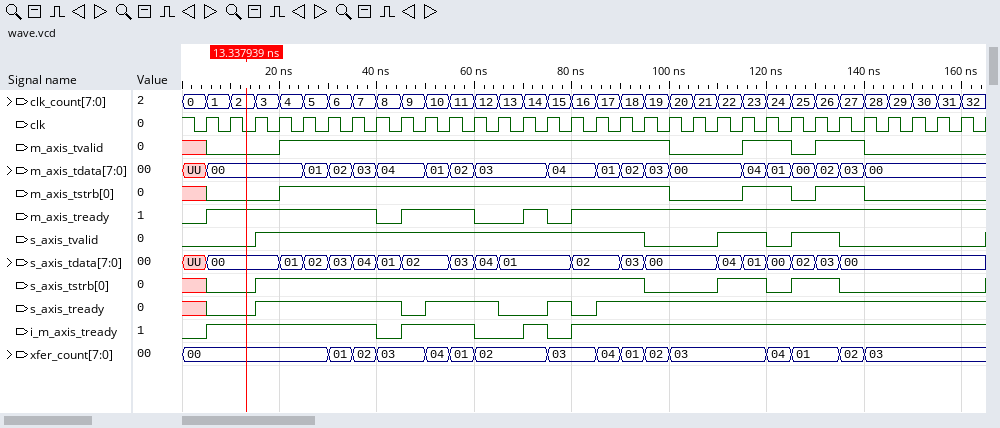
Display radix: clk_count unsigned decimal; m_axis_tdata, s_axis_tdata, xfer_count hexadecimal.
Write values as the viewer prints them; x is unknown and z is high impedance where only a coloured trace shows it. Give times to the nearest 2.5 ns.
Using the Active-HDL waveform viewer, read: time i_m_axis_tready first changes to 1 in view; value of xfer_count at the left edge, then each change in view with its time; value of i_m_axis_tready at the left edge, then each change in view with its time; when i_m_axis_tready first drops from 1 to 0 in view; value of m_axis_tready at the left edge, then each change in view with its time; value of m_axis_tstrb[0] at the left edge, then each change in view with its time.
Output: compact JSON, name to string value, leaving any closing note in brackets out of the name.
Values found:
{"time i_m_axis_tready first changes to 1 in view": "5 ns", "value of xfer_count at the left edge, then each change in view with its time": "00, 01 at 30 ns, 02 at 35 ns, 03 at 40 ns, 04 at 50 ns, 01 at 55 ns, 02 at 60 ns, 03 at 75 ns, 04 at 85 ns, 01 at 90 ns, 02 at 95 ns, 03 at 100 ns, 04 at 120 ns, 01 at 125 ns, 02 at 135 ns, 03 at 140 ns", "value of i_m_axis_tready at the left edge, then each change in view with its time": "0, 1 at 5 ns, 0 at 40 ns, 1 at 45 ns, 0 at 60 ns, 1 at 70 ns, 0 at 75 ns, 1 at 80 ns", "when i_m_axis_tready first drops from 1 to 0 in view": "40 ns", "value of m_axis_tready at the left edge, then each change in view with its time": "0, 1 at 5 ns, 0 at 40 ns, 1 at 45 ns, 0 at 60 ns, 1 at 70 ns, 0 at 75 ns, 1 at 80 ns", "value of m_axis_tstrb[0] at the left edge, then each change in view with its time": "x, 0 at 5 ns, 1 at 20 ns, 0 at 100 ns, 1 at 115 ns, 0 at 125 ns, 1 at 130 ns, 0 at 140 ns"}
